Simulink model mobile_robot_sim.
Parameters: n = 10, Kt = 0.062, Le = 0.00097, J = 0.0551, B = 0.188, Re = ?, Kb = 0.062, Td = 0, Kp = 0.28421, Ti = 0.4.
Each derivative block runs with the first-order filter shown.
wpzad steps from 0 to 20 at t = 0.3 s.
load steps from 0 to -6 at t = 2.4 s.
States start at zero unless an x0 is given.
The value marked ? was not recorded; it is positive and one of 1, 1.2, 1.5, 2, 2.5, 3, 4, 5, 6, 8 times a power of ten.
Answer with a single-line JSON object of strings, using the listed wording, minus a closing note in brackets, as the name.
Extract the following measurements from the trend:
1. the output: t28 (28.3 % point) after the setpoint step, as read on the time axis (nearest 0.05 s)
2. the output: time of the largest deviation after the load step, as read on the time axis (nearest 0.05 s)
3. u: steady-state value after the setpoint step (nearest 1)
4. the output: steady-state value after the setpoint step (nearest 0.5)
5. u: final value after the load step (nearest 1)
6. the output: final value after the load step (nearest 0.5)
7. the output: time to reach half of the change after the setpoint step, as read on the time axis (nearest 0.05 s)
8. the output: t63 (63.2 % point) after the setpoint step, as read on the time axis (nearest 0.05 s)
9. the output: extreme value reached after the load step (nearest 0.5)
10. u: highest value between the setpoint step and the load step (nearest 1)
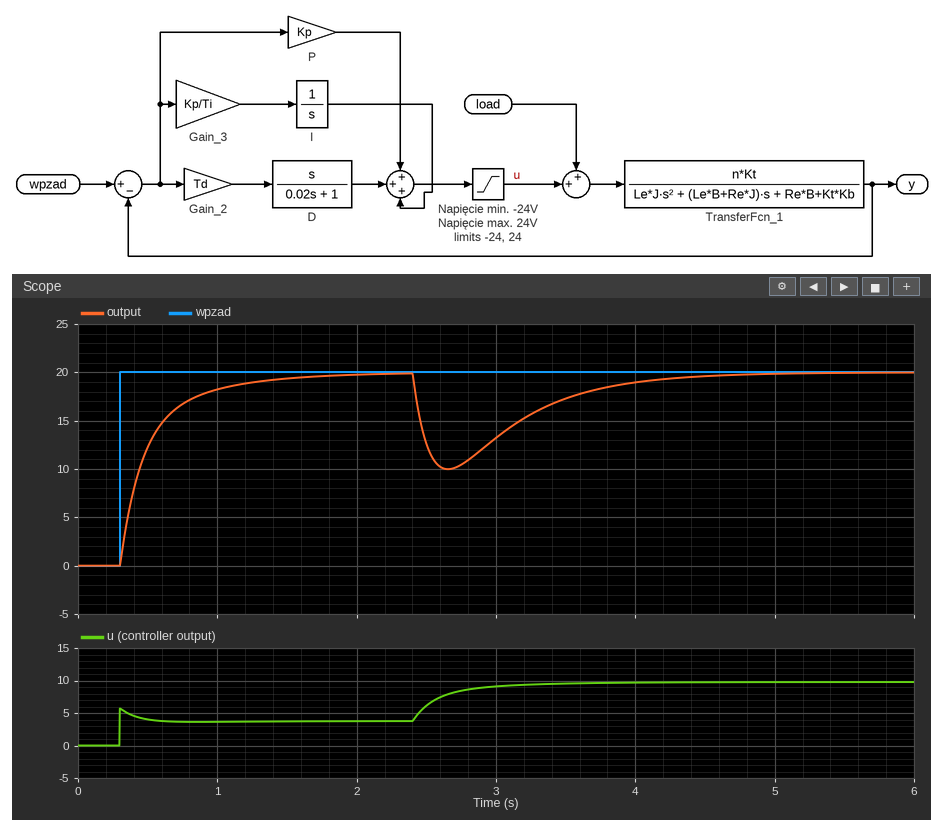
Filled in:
{"the output: t28 (28.3 % point) after the setpoint step, as read on the time axis": "0.35 s", "the output: time of the largest deviation after the load step, as read on the time axis": "2.65 s", "u: steady-state value after the setpoint step": "4", "the output: steady-state value after the setpoint step": "20.0", "u: final value after the load step": "10", "the output: final value after the load step": "20.0", "the output: time to reach half of the change after the setpoint step, as read on the time axis": "0.45 s", "the output: t63 (63.2 % point) after the setpoint step, as read on the time axis": "0.50 s", "the output: extreme value reached after the load step": "10.0", "u: highest value between the setpoint step and the load step": "6"}
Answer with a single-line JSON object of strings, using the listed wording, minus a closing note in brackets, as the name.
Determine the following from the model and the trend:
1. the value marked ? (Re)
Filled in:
{"the value marked ?": "0.6"}
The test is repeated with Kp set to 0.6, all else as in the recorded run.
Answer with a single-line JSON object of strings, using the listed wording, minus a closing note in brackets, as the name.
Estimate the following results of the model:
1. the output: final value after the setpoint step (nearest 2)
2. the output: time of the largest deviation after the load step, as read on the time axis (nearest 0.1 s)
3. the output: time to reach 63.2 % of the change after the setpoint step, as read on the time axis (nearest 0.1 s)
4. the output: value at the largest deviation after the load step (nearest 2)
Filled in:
{"the output: final value after the setpoint step": "20", "the output: time of the largest deviation after the load step, as read on the time axis": "2.6 s", "the output: time to reach 63.2 % of the change after the setpoint step, as read on the time axis": "0.4 s", "the output: value at the largest deviation after the load step": "14"}
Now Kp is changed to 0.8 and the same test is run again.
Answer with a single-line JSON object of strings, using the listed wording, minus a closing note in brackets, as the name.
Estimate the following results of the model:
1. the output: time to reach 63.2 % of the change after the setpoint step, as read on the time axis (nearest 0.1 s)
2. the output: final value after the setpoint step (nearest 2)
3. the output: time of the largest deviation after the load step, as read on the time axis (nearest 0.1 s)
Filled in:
{"the output: time to reach 63.2 % of the change after the setpoint step, as read on the time axis": "0.4 s", "the output: final value after the setpoint step": "20", "the output: time of the largest deviation after the load step, as read on the time axis": "2.5 s"}
